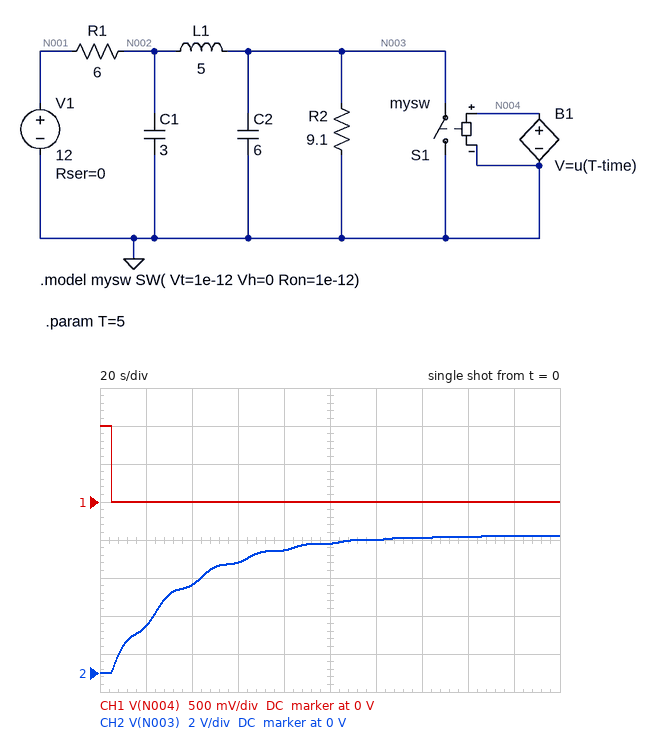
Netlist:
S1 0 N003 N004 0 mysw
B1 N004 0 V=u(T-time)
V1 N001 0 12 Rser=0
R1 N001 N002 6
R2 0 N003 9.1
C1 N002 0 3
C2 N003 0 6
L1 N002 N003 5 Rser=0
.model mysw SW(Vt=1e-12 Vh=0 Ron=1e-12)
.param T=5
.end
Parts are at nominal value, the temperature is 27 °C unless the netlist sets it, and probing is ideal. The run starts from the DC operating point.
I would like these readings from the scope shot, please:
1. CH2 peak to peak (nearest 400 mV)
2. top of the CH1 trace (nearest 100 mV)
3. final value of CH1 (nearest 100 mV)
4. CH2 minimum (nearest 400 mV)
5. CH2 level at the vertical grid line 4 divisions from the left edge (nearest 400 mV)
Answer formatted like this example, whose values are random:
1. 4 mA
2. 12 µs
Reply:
1. 7.2 V
2. 1.0 V
3. 0 V
4. 0 V
5. 6.4 V
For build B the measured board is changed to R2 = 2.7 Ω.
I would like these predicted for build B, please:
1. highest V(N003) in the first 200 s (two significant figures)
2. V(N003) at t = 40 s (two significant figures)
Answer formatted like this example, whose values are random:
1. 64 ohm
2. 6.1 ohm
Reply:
1. 3.7 V
2. 3.1 V
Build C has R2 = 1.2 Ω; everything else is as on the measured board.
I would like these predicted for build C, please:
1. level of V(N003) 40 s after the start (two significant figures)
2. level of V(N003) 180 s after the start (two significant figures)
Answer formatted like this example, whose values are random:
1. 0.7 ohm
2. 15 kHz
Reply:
1. 1.9 V
2. 2.0 V
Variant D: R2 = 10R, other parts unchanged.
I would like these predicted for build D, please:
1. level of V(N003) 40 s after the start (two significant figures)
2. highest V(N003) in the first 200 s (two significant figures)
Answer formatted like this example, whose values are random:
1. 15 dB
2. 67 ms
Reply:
1. 4.7 V
2. 7.5 V
